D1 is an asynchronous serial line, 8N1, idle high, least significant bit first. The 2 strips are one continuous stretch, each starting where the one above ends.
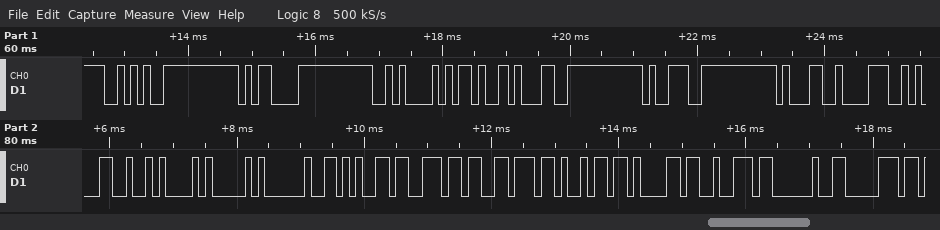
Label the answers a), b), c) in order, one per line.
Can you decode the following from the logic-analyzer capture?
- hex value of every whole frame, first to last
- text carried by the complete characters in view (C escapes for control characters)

a) 2A 0D 0A 2D 31 39 31 38 31 0A 41 20 65 6E 76 69 61 72 20 70
b) "*\r\n-19181\nA enviar p"
